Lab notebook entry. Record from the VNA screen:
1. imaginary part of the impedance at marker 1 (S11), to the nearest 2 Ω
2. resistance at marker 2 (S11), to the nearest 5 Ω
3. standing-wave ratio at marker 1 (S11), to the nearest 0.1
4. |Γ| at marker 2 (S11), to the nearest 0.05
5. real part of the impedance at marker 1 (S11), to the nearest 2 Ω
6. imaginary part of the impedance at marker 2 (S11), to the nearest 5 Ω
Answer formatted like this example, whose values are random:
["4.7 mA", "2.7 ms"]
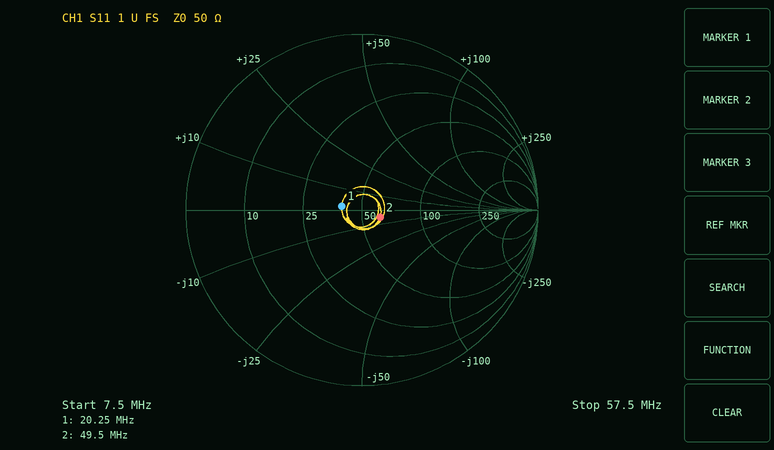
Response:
["+2 Ω", "60 Ω", "1.3", "0.10", "40 Ω", "-5 Ω"]
